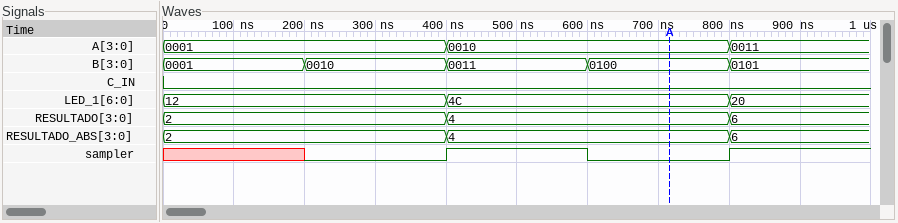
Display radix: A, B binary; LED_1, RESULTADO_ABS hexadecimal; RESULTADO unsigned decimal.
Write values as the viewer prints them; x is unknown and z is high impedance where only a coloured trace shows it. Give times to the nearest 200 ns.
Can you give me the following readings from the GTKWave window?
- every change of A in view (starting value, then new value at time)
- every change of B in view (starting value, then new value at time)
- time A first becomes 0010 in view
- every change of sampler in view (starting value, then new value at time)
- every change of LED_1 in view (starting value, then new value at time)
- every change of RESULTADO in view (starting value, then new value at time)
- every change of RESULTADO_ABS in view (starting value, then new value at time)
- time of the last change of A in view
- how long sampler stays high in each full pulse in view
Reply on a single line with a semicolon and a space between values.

0001, 0010 at 400 ns, 0011 at 800 ns; 0001, 0010 at 200 ns, 0011 at 400 ns, 0100 at 600 ns, 0101 at 800 ns; 400 ns; x, 0 at 200 ns, 1 at 400 ns, 0 at 600 ns, 1 at 800 ns; 12, 4C at 400 ns, 20 at 800 ns; 2, 4 at 400 ns, 6 at 800 ns; 2, 4 at 400 ns, 6 at 800 ns; 800 ns; 200 ns
